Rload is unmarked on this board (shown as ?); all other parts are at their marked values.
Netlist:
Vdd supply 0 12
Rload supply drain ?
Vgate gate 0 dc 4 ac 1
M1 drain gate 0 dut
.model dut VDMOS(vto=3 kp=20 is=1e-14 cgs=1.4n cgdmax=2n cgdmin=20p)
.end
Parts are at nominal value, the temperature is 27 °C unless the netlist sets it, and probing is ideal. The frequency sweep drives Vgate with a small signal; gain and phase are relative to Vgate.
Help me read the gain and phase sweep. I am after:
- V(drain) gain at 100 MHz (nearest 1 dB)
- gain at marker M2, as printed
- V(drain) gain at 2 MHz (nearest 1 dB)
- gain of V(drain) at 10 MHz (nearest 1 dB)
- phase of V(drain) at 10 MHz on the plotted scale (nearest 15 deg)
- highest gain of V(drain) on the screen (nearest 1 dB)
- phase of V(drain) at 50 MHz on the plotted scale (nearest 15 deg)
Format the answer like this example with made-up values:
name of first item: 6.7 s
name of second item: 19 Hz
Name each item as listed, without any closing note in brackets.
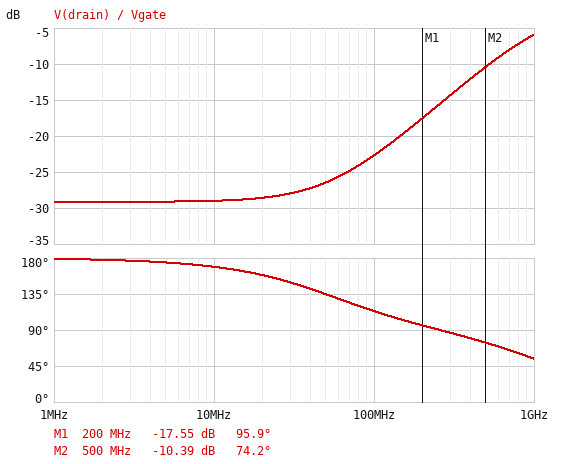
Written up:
V(drain) gain at 100 MHz: -23 dB
gain at marker M2, as printed: -10.39 dB
V(drain) gain at 2 MHz: -29 dB
gain of V(drain) at 10 MHz: -29 dB
phase of V(drain) at 10 MHz on the plotted scale: 165 deg
highest gain of V(drain) on the screen: -6 dB
phase of V(drain) at 50 MHz on the plotted scale: 135 deg
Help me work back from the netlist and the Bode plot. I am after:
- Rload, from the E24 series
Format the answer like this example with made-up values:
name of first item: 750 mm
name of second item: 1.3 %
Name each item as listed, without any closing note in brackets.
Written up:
Rload, from the E24 series: 18 Ω
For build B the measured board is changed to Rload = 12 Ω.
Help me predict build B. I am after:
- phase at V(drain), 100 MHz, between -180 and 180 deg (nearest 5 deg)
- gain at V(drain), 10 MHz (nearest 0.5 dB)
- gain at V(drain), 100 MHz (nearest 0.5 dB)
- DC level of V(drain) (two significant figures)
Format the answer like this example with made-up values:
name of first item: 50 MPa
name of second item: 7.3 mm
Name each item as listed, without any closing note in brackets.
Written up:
phase at V(drain), 100 MHz, between -180 and 180 deg: 125 deg
gain at V(drain), 10 MHz: -25.5 dB
gain at V(drain), 100 MHz: -21.5 dB
DC level of V(drain): 51 mV
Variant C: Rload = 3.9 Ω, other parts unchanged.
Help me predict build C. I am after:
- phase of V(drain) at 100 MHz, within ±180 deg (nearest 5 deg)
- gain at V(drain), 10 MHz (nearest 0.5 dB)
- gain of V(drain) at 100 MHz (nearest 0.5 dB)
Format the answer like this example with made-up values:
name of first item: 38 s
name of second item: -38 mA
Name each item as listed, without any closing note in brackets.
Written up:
phase of V(drain) at 100 MHz, within ±180 deg: 155 deg
gain at V(drain), 10 MHz: -14.0 dB
gain of V(drain) at 100 MHz: -13.5 dB
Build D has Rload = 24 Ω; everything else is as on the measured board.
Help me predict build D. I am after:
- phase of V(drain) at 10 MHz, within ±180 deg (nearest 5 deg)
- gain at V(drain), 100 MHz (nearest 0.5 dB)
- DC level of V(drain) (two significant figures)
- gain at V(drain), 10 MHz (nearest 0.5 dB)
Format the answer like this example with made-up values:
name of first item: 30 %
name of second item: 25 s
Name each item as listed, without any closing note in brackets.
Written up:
phase of V(drain) at 10 MHz, within ±180 deg: 165 deg
gain at V(drain), 100 MHz: -23.0 dB
DC level of V(drain): 25 mV
gain at V(drain), 10 MHz: -31.5 dB
